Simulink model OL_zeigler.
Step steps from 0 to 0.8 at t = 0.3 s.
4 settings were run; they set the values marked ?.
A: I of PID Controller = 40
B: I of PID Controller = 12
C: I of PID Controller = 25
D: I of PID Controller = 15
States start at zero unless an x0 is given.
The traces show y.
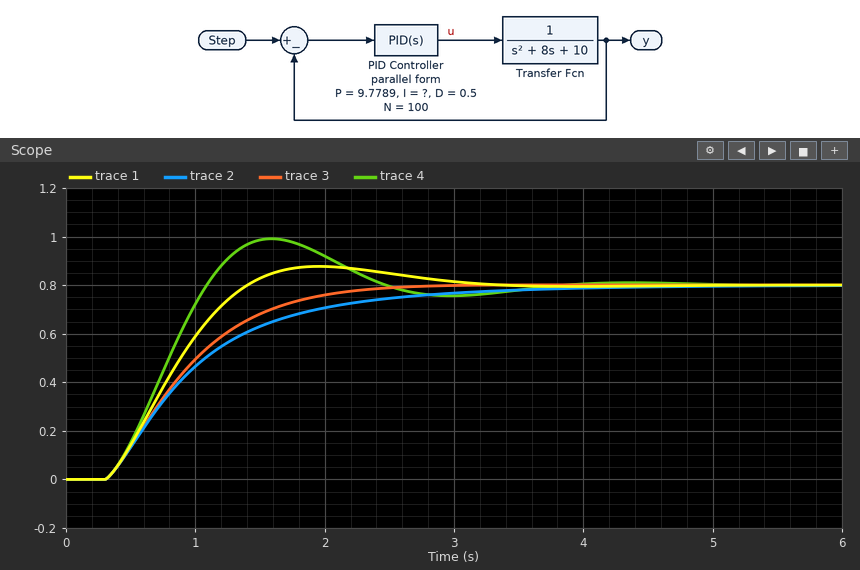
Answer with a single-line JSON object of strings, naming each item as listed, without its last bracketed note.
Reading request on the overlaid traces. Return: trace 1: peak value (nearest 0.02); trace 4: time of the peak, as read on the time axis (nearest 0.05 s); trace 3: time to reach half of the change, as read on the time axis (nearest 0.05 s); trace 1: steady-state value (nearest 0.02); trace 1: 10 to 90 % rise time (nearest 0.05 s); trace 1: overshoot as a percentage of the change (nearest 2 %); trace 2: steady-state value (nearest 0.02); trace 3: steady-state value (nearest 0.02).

{"trace 1: peak value": "0.88", "trace 4: time of the peak, as read on the time axis": "1.60 s", "trace 3: time to reach half of the change, as read on the time axis": "0.85 s", "trace 1: steady-state value": "0.80", "trace 1: 10 to 90 % rise time": "0.80 s", "trace 1: overshoot as a percentage of the change": "10 %", "trace 2: steady-state value": "0.80", "trace 3: steady-state value": "0.80"}
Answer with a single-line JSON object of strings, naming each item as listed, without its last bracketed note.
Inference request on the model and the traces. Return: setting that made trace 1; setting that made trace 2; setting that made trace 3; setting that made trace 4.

{"setting that made trace 1": "C", "setting that made trace 2": "B", "setting that made trace 3": "D", "setting that made trace 4": "A"}
